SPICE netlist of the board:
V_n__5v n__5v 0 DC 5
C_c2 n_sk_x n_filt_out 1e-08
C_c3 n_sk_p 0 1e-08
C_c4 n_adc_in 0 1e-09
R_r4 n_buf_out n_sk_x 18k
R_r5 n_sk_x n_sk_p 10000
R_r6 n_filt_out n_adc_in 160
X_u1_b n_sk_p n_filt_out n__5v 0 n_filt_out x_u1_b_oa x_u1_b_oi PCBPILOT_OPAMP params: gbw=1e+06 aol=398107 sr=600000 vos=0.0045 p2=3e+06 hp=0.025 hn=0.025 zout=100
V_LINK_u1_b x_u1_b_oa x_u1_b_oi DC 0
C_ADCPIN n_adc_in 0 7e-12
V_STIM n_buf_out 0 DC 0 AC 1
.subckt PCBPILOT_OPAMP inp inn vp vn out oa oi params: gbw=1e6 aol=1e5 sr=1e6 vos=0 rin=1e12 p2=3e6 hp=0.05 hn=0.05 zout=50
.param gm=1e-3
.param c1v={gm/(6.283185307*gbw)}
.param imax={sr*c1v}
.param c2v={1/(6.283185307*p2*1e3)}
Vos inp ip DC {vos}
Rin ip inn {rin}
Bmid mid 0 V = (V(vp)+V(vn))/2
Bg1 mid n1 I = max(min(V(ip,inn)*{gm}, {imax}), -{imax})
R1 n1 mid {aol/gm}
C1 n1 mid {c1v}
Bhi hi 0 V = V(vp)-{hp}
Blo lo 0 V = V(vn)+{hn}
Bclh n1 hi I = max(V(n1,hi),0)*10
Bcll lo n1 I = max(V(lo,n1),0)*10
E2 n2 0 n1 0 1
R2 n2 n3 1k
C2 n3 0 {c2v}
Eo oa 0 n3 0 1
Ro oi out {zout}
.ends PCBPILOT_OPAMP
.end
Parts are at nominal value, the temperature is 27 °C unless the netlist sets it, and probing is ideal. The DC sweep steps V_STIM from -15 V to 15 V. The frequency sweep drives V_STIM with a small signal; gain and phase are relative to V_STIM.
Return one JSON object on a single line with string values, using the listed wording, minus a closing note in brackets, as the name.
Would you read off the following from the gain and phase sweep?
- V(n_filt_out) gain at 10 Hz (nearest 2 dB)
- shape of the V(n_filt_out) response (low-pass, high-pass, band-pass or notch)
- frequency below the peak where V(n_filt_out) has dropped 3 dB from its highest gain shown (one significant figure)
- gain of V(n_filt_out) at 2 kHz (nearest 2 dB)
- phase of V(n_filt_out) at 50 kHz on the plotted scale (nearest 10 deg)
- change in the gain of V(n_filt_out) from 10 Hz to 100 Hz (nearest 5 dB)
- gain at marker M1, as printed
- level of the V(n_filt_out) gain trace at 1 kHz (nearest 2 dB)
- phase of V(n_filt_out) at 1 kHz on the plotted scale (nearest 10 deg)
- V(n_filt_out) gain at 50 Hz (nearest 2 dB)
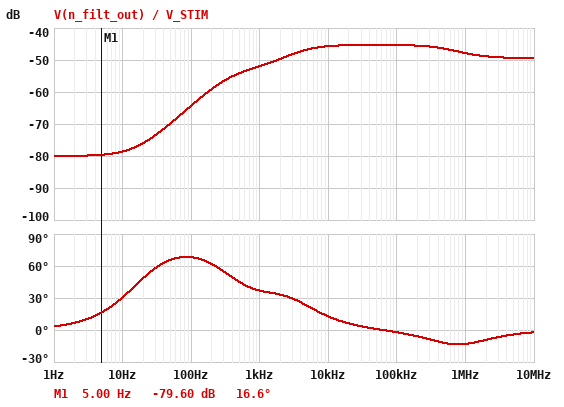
{"V(n_filt_out) gain at 10 Hz": "-78 dB", "shape of the V(n_filt_out) response": "high-pass", "frequency below the peak where V(n_filt_out) has dropped 3 dB from its highest gain shown": "3 kHz", "gain of V(n_filt_out) at 2 kHz": "-50 dB", "phase of V(n_filt_out) at 50 kHz on the plotted scale": "0 deg", "change in the gain of V(n_filt_out) from 10 Hz to 100 Hz": "15 dB", "gain at marker M1, as printed": "-79.60 dB", "level of the V(n_filt_out) gain trace at 1 kHz": "-52 dB", "phase of V(n_filt_out) at 1 kHz on the plotted scale": "40 deg", "V(n_filt_out) gain at 50 Hz": "-70 dB"}
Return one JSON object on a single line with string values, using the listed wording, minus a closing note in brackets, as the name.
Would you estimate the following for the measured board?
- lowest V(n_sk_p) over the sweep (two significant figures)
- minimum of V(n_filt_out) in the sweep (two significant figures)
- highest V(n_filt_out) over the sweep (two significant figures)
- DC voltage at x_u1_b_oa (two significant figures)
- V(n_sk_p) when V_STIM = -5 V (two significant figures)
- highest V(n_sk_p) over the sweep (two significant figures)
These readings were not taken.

{"lowest V(n_sk_p) over the sweep": "-15 V", "minimum of V(n_filt_out) in the sweep": "25 mV", "highest V(n_filt_out) over the sweep": "5.0 V", "DC voltage at x_u1_b_oa": "25 mV", "V(n_sk_p) when V_STIM = -5 V": "-5.0 V", "highest V(n_sk_p) over the sweep": "15 V"}
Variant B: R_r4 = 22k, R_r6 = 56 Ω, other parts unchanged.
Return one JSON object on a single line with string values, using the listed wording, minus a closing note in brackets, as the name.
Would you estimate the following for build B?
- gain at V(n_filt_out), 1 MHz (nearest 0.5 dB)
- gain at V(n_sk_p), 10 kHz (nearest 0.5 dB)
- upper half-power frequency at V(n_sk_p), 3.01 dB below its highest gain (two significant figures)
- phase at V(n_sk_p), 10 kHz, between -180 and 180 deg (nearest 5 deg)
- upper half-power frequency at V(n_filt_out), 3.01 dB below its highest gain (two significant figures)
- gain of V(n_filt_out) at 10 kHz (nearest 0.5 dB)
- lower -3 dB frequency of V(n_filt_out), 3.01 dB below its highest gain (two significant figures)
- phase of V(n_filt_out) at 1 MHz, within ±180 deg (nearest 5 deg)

{"gain at V(n_filt_out), 1 MHz": "-49.5 dB", "gain at V(n_sk_p), 10 kHz": "-39.5 dB", "upper half-power frequency at V(n_sk_p), 3.01 dB below its highest gain": "320 Hz", "phase at V(n_sk_p), 10 kHz, between -180 and 180 deg": "-155 deg", "upper half-power frequency at V(n_filt_out), 3.01 dB below its highest gain": "1.2 MHz", "gain of V(n_filt_out) at 10 kHz": "-47.5 dB", "lower -3 dB frequency of V(n_filt_out), 3.01 dB below its highest gain": "2.8 kHz", "phase of V(n_filt_out) at 1 MHz, within ±180 deg": "-25 deg"}
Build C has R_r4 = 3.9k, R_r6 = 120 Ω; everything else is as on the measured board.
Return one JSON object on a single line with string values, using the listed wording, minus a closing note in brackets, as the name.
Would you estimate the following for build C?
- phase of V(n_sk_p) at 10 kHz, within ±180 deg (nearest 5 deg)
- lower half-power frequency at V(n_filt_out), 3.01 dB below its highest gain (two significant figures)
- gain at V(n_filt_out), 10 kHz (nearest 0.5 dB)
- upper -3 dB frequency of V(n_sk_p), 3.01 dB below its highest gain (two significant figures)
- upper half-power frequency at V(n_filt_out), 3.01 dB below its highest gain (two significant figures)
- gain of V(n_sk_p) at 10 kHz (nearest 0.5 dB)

{"phase of V(n_sk_p) at 10 kHz, within ±180 deg": "-140 deg", "lower half-power frequency at V(n_filt_out), 3.01 dB below its highest gain": "5.7 kHz", "gain at V(n_filt_out), 10 kHz": "-33.5 dB", "upper -3 dB frequency of V(n_sk_p), 3.01 dB below its highest gain": "1.0 kHz", "upper half-power frequency at V(n_filt_out), 3.01 dB below its highest gain": "1.2 MHz", "gain of V(n_sk_p) at 10 kHz": "-25.5 dB"}
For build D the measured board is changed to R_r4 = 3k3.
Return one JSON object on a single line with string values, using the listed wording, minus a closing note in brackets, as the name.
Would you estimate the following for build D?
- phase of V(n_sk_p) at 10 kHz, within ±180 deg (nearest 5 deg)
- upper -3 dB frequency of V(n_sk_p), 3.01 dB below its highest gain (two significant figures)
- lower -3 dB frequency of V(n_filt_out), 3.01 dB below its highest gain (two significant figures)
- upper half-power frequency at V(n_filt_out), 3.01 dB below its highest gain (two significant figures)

{"phase of V(n_sk_p) at 10 kHz, within ±180 deg": "-135 deg", "upper -3 dB frequency of V(n_sk_p), 3.01 dB below its highest gain": "1.1 kHz", "lower -3 dB frequency of V(n_filt_out), 3.01 dB below its highest gain": "6.3 kHz", "upper half-power frequency at V(n_filt_out), 3.01 dB below its highest gain": "1.4 MHz"}
